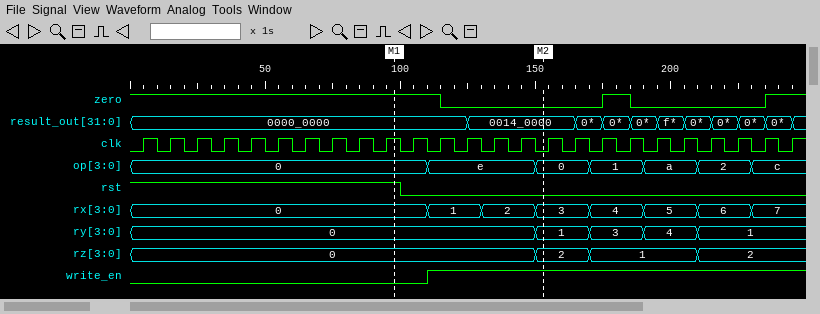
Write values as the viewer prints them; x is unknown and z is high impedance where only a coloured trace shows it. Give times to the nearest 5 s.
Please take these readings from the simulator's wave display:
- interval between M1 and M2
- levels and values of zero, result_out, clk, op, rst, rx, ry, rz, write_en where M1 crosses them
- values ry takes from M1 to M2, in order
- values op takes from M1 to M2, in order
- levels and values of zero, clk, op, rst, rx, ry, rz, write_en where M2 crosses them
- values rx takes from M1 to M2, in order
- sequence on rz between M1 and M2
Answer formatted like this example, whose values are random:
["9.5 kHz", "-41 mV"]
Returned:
["55 s", "zero=1, result_out=0000_0000, clk=1, op=0, rst=1, rx=0, ry=0, rz=0, write_en=0", "0, 1", "0, e, 0", "zero=0, clk=0, op=0, rst=0, rx=3, ry=1, rz=2, write_en=1", "0, 1, 2, 3", "0, 2"]
